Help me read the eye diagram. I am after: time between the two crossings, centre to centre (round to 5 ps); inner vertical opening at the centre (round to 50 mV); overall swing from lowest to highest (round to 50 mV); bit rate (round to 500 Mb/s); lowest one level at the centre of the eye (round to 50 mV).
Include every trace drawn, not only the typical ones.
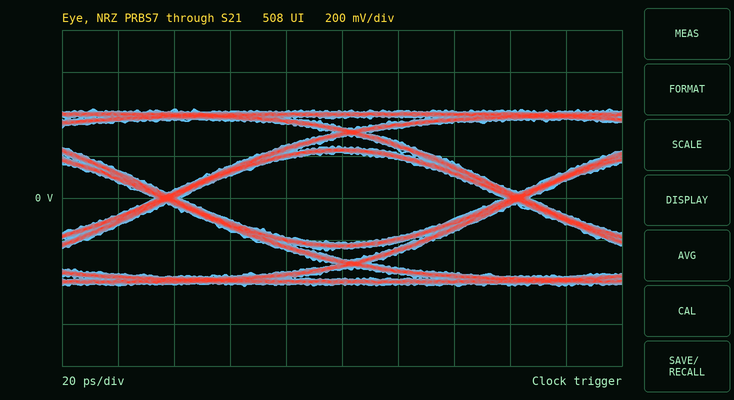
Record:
125 ps
450 mV
850 mV
8.0 Gb/s
200 mV
